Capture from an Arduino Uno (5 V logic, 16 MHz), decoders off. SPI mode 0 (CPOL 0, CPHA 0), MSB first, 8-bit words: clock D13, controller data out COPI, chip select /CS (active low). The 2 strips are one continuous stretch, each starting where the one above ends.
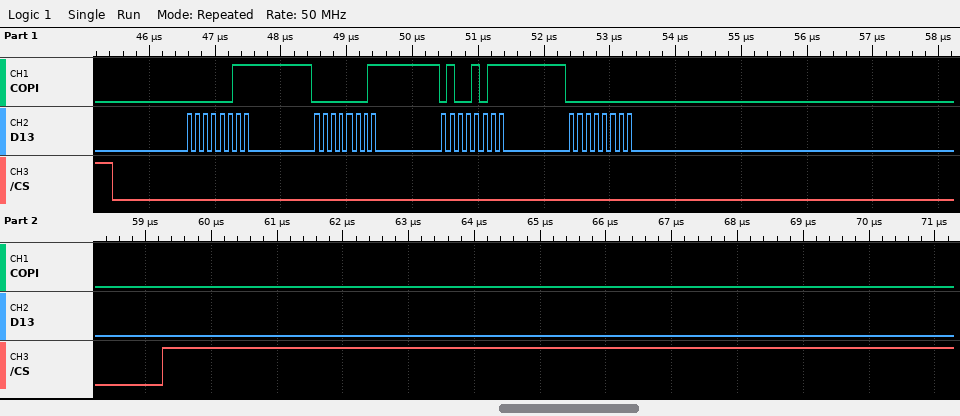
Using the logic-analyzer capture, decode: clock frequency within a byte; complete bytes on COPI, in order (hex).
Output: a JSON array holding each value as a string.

["8 MHz", "03 01 4B 00"]
